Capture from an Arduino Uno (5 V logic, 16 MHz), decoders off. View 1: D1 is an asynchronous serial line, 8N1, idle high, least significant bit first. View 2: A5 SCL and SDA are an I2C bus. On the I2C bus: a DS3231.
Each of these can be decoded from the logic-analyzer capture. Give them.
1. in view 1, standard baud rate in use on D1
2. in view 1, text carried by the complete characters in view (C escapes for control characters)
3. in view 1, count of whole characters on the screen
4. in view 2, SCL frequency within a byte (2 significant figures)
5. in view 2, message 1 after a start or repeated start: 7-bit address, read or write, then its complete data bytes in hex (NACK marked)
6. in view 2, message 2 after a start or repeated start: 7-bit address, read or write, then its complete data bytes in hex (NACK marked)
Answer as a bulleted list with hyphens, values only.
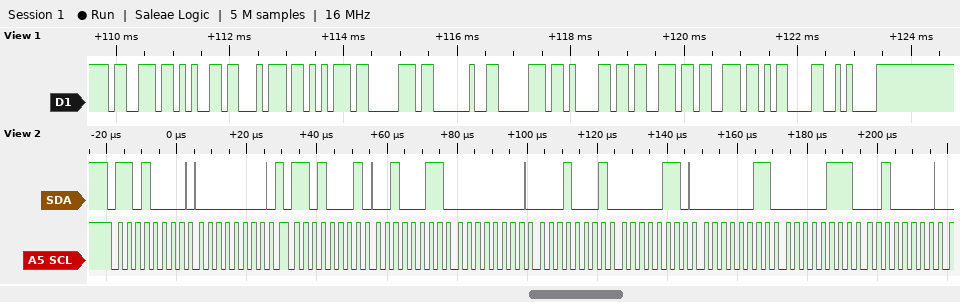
- 9600 baud
- "setup pass\r\n"
- 12
- 400 kHz
- 0x68 write: 00
- 0x68 read: 23 00 11 06 03 07 20
